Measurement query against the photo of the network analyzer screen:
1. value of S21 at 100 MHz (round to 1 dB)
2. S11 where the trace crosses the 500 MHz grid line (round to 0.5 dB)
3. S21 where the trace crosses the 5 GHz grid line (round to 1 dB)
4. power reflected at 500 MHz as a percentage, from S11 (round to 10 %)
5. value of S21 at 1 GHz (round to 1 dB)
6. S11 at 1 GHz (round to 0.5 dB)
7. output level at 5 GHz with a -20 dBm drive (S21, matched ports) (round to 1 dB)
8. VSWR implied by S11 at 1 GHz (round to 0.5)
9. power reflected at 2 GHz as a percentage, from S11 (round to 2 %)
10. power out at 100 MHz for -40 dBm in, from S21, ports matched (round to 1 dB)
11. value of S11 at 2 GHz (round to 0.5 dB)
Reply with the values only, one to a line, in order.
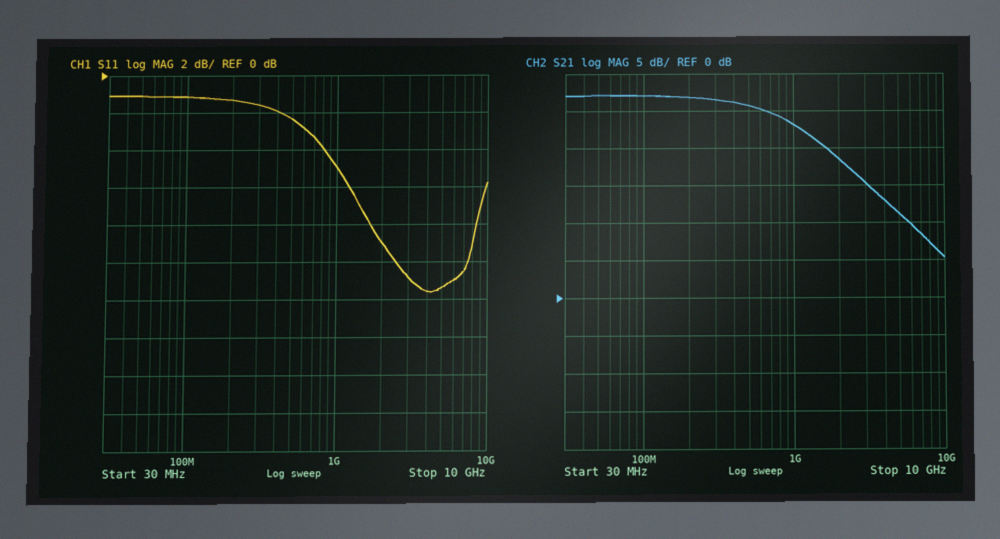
27 dB
-2.5 dB
11 dB
60 %
23 dB
-5.0 dB
-9 dBm
3.5
12 %
-13 dBm
-9.0 dB
